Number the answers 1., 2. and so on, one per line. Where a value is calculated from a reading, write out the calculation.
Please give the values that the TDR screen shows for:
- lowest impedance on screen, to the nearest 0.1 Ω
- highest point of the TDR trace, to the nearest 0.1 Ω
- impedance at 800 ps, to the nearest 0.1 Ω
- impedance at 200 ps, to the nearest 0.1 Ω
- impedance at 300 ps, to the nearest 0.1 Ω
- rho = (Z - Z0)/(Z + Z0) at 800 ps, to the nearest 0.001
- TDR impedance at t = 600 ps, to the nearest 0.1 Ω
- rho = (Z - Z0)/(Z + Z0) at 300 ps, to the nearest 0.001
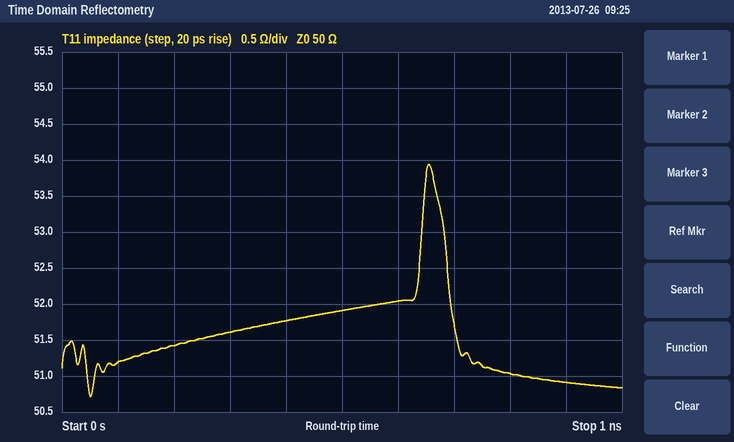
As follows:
1. 50.7 Ω
2. 53.9 Ω
3. 51.0 Ω
4. 51.4 Ω
5. 51.6 Ω
6. (51 − 50)/(51 + 50) ≈ +0.010
7. 52.0 Ω
8. (51.6 − 50)/(51.6 + 50) ≈ +0.016
